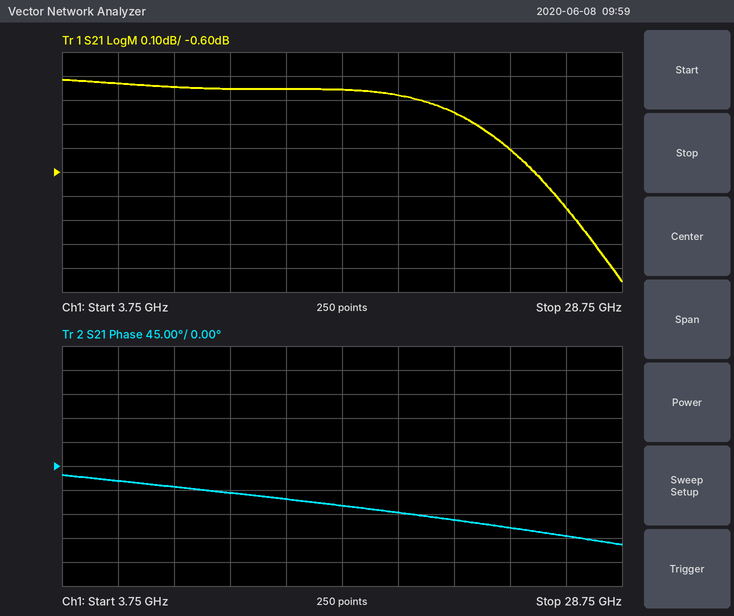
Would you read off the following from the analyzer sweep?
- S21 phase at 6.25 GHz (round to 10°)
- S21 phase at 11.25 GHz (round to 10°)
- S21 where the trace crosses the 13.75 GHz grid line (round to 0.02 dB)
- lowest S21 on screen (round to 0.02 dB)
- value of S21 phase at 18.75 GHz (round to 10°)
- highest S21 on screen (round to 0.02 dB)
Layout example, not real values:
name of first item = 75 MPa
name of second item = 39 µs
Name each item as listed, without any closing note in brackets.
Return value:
S21 phase at 6.25 GHz = -30°
S21 phase at 11.25 GHz = -50°
S21 where the trace crosses the 13.75 GHz grid line = -0.26 dB
lowest S21 on screen = -1.06 dB
value of S21 phase at 18.75 GHz = -90°
highest S21 on screen = -0.22 dB
